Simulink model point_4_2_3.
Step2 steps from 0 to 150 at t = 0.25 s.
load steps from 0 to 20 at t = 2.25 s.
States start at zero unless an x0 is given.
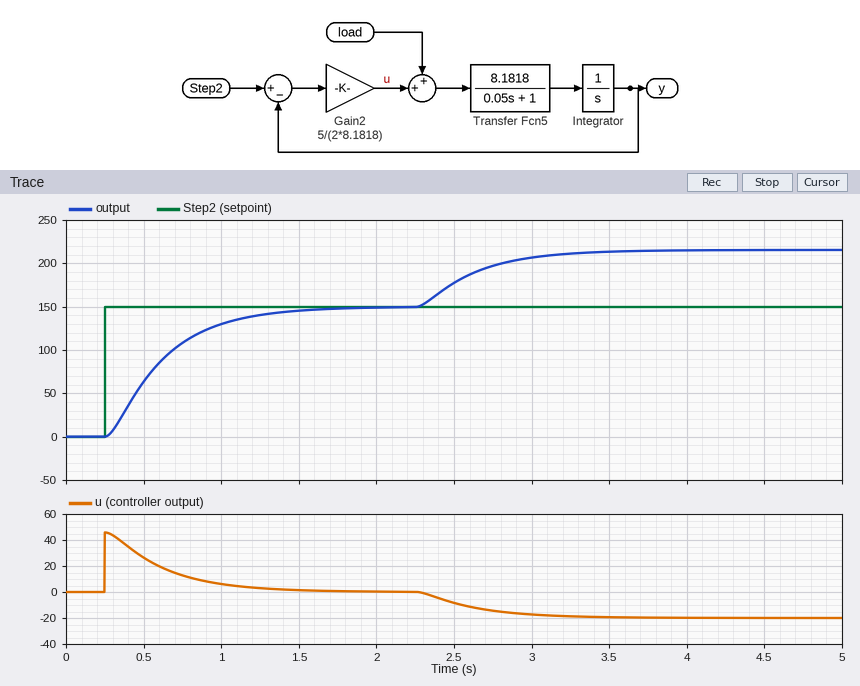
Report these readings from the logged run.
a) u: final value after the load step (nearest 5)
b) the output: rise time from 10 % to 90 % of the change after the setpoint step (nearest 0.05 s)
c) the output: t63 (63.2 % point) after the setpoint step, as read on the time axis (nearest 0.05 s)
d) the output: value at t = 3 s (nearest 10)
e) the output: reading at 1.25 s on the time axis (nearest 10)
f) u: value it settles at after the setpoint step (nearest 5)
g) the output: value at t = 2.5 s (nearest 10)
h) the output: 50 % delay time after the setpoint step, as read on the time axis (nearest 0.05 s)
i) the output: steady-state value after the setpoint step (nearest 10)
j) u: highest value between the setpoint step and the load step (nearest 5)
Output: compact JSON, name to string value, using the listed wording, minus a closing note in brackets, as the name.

{"u: final value after the load step": "-20", "the output: rise time from 10 % to 90 % of the change after the setpoint step": "0.75 s", "the output: t63 (63.2 % point) after the setpoint step, as read on the time axis": "0.65 s", "the output: value at t = 3 s": "210", "the output: reading at 1.25 s on the time axis": "140", "u: value it settles at after the setpoint step": "0", "the output: value at t = 2.5 s": "180", "the output: 50 % delay time after the setpoint step, as read on the time axis": "0.55 s", "the output: steady-state value after the setpoint step": "150", "u: highest value between the setpoint step and the load step": "45"}
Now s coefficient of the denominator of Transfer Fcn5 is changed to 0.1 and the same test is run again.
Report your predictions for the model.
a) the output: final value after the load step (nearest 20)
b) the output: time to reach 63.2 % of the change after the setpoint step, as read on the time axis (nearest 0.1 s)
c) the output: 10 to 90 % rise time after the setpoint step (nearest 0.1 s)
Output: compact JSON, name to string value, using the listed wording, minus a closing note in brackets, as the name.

{"the output: final value after the load step": "220", "the output: time to reach 63.2 % of the change after the setpoint step, as read on the time axis": "0.7 s", "the output: 10 to 90 % rise time after the setpoint step": "0.7 s"}
